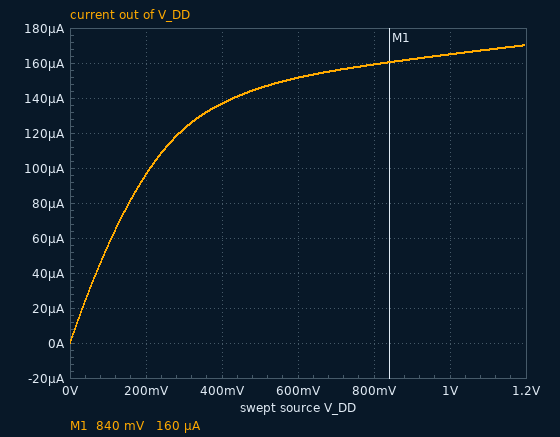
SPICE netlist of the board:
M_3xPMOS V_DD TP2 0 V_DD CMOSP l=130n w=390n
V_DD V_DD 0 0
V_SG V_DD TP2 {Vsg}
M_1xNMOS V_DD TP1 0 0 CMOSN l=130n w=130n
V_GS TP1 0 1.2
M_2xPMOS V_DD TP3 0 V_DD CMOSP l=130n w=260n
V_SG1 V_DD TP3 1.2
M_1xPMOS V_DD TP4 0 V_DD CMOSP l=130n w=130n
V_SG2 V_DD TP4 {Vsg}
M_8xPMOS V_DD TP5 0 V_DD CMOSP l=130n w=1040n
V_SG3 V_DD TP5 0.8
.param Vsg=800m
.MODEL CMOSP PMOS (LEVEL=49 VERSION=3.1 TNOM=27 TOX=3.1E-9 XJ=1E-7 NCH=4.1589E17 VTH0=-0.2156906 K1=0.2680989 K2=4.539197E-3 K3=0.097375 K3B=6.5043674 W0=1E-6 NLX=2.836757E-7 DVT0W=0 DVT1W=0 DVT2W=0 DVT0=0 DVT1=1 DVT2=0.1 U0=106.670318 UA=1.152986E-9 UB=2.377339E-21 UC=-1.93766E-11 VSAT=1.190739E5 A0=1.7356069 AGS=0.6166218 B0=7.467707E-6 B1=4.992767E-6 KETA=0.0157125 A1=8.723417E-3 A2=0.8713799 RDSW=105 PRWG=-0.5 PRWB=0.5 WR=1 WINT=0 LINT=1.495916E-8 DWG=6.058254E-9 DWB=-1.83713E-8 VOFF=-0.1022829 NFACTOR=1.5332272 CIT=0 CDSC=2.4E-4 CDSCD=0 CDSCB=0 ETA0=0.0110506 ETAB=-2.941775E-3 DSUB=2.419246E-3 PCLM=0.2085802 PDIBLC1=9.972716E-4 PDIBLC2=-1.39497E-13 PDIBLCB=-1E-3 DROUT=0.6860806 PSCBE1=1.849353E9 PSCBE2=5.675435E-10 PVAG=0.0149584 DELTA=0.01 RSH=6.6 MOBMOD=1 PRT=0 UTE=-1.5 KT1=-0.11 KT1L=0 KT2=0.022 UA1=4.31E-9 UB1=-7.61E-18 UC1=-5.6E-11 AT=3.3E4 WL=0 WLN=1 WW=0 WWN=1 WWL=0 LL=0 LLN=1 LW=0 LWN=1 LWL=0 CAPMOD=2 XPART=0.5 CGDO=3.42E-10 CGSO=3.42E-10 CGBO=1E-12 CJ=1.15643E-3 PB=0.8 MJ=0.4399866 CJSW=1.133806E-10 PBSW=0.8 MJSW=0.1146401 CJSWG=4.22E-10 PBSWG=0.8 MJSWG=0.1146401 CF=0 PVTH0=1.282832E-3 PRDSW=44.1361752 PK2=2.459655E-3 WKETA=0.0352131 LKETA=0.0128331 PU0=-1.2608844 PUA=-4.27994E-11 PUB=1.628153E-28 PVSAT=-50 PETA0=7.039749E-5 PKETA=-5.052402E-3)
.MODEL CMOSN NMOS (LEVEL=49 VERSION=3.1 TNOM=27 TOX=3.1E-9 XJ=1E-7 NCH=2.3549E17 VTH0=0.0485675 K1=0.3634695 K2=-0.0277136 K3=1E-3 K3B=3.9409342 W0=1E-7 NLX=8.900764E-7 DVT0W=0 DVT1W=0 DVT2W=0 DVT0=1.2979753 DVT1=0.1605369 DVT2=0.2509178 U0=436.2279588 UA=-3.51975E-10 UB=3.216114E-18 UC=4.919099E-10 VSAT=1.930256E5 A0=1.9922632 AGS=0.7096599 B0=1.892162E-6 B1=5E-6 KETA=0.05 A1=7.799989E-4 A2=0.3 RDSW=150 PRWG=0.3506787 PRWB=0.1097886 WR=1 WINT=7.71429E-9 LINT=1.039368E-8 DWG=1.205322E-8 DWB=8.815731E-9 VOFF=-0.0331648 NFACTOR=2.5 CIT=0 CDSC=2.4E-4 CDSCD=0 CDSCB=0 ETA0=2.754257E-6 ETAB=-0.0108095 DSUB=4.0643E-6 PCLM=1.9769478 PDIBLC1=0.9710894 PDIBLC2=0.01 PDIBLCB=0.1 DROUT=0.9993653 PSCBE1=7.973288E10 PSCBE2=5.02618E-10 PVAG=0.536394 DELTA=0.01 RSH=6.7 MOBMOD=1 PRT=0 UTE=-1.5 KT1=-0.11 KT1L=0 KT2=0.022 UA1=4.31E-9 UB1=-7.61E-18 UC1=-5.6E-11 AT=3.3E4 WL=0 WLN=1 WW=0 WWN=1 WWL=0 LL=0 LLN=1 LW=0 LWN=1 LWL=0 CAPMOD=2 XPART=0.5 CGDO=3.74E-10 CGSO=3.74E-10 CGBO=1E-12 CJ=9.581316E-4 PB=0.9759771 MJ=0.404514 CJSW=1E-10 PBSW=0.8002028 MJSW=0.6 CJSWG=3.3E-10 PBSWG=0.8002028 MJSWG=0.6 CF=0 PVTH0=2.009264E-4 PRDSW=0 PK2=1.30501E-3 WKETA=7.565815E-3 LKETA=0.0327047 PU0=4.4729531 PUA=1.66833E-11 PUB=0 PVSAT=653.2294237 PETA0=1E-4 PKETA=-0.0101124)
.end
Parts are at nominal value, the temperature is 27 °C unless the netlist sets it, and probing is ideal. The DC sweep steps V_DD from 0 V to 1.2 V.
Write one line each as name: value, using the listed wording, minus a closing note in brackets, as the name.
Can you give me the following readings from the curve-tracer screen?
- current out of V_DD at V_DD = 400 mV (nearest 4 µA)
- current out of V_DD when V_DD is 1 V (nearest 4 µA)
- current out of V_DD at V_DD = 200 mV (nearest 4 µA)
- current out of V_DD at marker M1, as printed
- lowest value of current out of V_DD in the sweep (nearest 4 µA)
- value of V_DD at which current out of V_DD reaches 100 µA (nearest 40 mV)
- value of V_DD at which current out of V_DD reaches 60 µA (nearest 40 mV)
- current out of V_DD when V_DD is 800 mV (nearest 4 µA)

current out of V_DD at V_DD = 400 mV: 136 µA
current out of V_DD when V_DD is 1 V: 164 µA
current out of V_DD at V_DD = 200 mV: 96 µA
current out of V_DD at marker M1, as printed: 160 µA
lowest value of current out of V_DD in the sweep: 0 A
value of V_DD at which current out of V_DD reaches 100 µA: 200 mV
value of V_DD at which current out of V_DD reaches 60 µA: 120 mV
current out of V_DD when V_DD is 800 mV: 160 µA
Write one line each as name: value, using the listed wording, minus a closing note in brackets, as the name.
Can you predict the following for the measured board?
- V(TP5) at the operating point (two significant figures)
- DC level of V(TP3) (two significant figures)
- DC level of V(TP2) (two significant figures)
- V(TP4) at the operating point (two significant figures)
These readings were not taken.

V(TP5) at the operating point: -800 mV
DC level of V(TP3): -1.2 V
DC level of V(TP2): -800 mV
V(TP4) at the operating point: -800 mV
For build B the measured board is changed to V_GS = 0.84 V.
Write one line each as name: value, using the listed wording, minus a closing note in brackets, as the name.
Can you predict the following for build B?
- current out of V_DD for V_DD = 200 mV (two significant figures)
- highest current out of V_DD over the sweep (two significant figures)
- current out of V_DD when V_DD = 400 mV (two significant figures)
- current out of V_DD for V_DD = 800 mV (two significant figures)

current out of V_DD for V_DD = 200 mV: 87 µA
highest current out of V_DD over the sweep: 150 µA
current out of V_DD when V_DD = 400 mV: 120 µA
current out of V_DD for V_DD = 800 mV: 140 µA
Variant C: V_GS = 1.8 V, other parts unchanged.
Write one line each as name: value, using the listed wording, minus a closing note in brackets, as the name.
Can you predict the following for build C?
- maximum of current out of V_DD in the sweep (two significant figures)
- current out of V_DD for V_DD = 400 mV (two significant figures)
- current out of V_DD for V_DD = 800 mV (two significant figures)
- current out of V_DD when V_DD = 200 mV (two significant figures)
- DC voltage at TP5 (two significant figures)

maximum of current out of V_DD in the sweep: 190 µA
current out of V_DD for V_DD = 400 mV: 150 µA
current out of V_DD for V_DD = 800 mV: 180 µA
current out of V_DD when V_DD = 200 mV: 99 µA
DC voltage at TP5: -800 mV
